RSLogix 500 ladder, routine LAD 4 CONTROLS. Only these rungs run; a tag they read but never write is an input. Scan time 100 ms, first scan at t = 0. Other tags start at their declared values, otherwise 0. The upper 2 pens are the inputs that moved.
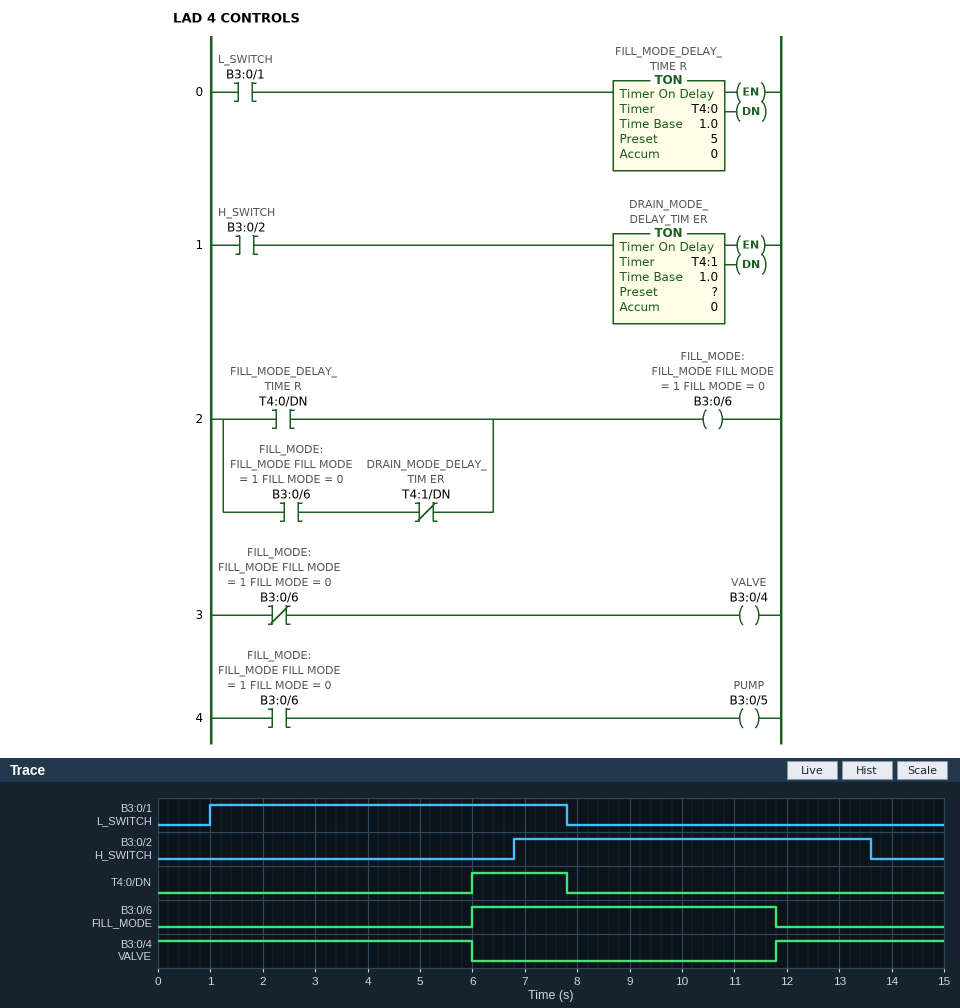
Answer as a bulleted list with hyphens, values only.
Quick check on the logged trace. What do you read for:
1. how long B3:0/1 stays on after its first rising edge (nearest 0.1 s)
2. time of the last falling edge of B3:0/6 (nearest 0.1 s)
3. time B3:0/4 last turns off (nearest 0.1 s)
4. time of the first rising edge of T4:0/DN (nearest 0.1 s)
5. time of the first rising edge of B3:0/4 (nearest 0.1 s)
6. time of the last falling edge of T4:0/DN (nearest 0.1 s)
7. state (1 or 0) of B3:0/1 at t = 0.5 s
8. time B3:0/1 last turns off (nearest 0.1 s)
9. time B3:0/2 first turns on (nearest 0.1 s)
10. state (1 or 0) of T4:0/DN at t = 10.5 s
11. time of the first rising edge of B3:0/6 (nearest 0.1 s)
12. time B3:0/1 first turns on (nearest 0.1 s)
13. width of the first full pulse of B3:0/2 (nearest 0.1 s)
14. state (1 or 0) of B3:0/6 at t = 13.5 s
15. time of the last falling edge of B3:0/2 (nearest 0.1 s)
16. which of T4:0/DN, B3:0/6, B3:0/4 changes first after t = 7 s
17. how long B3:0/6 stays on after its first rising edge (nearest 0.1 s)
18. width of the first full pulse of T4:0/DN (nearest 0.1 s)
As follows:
- 6.8 s
- 11.8 s
- 6.0 s
- 6.0 s
- 11.8 s
- 7.8 s
- 0
- 7.8 s
- 6.8 s
- 0
- 6.0 s
- 1.0 s
- 6.8 s
- 0
- 13.6 s
- T4:0/DN
- 5.8 s
- 1.8 s
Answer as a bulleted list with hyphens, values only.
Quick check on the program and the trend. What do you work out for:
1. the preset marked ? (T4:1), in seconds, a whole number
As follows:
- 5 s
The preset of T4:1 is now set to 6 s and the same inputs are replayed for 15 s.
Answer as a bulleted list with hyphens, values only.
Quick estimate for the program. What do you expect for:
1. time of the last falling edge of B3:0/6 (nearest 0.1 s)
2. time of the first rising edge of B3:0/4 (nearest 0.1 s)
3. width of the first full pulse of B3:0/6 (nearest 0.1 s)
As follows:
- 12.8 s
- 12.8 s
- 6.8 s
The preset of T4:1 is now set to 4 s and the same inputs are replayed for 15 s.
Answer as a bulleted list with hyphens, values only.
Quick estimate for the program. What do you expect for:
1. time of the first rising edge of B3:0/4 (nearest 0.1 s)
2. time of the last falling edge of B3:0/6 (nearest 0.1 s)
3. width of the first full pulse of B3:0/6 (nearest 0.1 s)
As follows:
- 10.8 s
- 10.8 s
- 4.8 s
